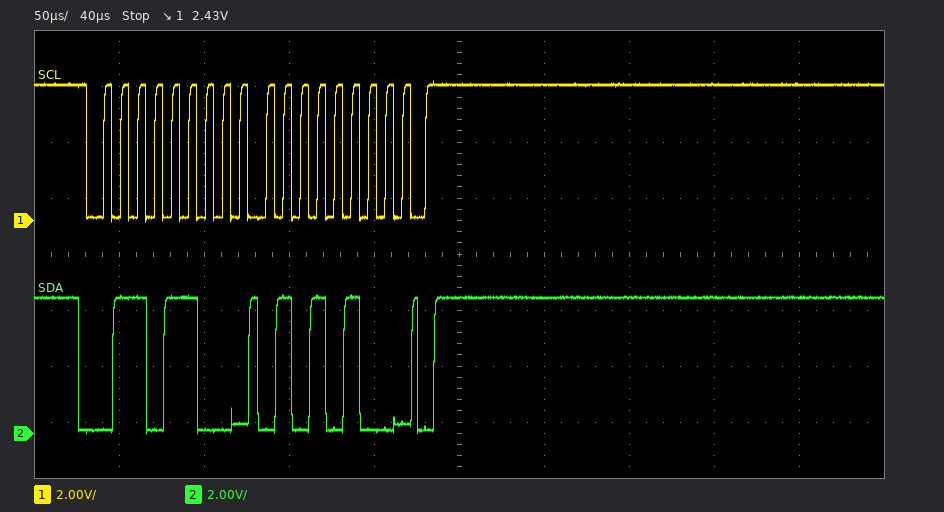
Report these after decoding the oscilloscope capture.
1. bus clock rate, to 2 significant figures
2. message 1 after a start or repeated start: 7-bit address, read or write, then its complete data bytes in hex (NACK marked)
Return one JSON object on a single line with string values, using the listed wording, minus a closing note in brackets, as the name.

{"bus clock rate, to 2 significant figures": "100 kHz", "message 1 after a start or repeated start: 7-bit address, read or write, then its complete data bytes in hex": "0x36 write: 54"}
